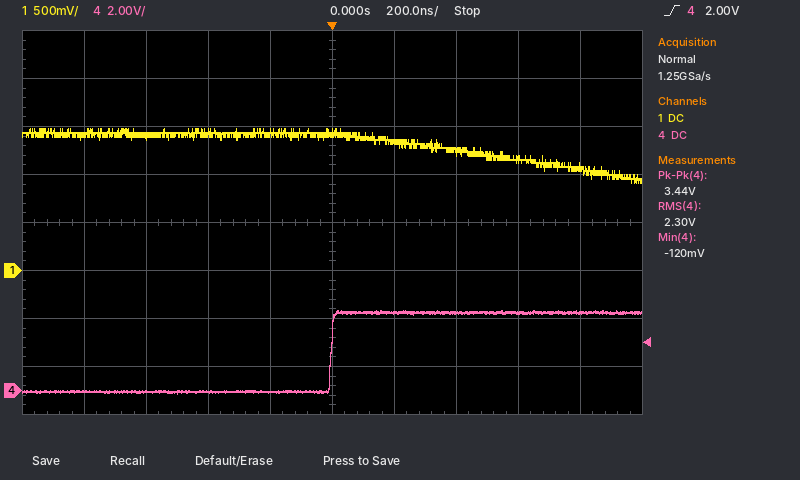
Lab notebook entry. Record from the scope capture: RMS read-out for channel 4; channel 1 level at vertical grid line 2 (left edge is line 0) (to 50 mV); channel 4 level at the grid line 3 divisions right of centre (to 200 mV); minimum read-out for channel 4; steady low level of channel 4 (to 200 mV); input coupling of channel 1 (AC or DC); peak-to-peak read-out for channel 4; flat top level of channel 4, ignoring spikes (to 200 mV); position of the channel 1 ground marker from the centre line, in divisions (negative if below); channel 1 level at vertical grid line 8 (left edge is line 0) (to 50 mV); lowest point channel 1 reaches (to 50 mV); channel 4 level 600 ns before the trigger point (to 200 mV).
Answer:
2.30 V
1.40 V
3.2 V
-120 mV
0.0 V
DC
3.44 V
3.2 V
-1.0 div
1.15 V
900 mV
0.0 V
